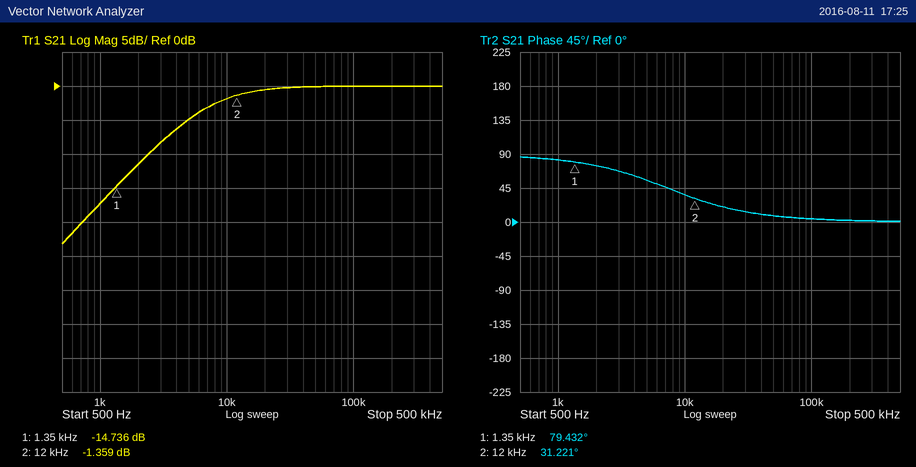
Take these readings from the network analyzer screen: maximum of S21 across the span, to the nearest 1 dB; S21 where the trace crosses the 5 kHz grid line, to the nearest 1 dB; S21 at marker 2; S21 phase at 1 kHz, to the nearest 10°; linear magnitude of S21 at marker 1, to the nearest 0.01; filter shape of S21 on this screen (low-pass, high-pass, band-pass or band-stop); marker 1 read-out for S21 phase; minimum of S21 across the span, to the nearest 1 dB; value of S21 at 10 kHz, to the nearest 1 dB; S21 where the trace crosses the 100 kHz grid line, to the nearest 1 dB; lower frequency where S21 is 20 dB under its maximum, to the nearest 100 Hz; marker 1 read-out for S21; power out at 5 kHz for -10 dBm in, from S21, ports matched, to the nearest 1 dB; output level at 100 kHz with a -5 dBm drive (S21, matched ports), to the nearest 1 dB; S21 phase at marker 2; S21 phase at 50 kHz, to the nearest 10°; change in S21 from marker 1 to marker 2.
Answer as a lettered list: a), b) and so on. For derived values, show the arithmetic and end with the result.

a) 0 dB
b) -5 dB
c) -1.359 dB
d) 80°
e) 10^(-14.736/20) ≈ 0.18
f) high-pass
g) 79.432°
h) -23 dB
i) -2 dB
j) 0 dB
k) 700 Hz
l) -14.736 dB
m) -10 dBm + (-5 dB) = -15 dBm
n) -5 dBm + (0 dB) = -5 dBm
o) 31.221°
p) 10°
q) -1.359 − (-14.736) = 13.377 dB
